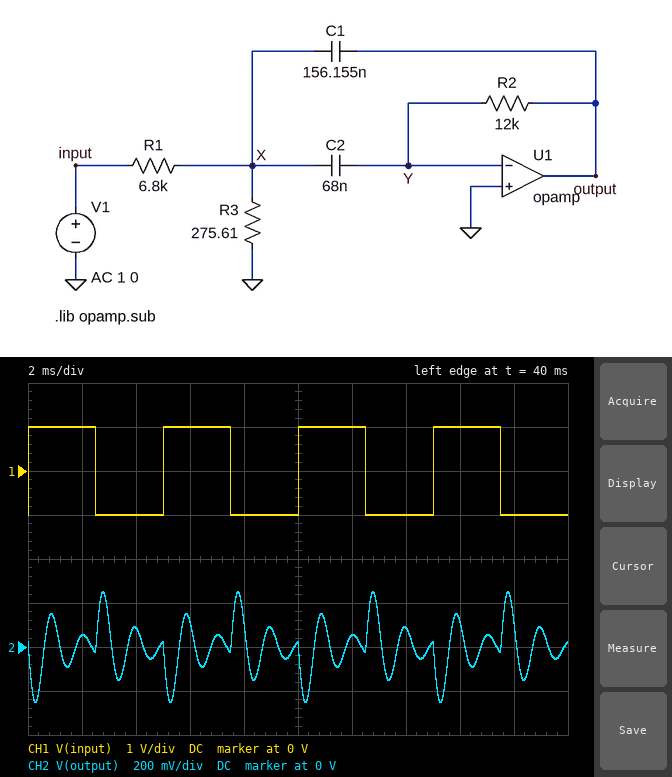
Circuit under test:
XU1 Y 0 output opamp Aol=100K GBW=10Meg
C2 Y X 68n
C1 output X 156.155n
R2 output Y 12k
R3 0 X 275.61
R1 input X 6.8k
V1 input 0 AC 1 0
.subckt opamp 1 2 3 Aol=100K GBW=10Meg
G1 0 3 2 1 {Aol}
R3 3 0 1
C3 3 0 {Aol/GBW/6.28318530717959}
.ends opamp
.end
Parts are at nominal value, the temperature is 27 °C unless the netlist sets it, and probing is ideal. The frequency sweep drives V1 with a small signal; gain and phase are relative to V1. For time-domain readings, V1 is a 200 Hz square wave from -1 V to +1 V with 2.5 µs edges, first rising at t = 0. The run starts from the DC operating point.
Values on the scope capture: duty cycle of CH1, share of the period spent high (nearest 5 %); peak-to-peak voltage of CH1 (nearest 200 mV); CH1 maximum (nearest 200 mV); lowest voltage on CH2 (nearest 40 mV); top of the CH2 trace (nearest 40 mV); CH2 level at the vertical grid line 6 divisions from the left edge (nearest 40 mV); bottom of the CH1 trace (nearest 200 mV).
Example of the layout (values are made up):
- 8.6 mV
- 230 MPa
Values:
- 50 %
- 2.0 V
- 1.0 V
- -240 mV
- 240 mV
- 40 mV
- -1.0 V
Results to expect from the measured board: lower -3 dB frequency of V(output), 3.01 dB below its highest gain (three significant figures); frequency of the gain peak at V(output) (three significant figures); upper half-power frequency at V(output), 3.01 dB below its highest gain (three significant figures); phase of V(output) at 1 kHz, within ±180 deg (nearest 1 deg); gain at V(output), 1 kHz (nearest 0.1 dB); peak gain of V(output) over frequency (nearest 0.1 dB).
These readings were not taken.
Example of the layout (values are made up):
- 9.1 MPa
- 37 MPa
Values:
- 737 Hz
- 866 Hz
- 1.02 kHz
- 138 deg
- -8.0 dB
- -5.4 dB
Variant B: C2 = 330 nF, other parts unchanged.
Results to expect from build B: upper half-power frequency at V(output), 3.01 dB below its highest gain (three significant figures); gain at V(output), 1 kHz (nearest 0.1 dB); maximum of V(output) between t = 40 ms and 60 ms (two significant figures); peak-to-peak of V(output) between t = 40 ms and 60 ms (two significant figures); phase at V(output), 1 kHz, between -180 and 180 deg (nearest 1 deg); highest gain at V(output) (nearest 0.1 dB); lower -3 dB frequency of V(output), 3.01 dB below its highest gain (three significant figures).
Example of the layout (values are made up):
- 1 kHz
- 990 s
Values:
- 461 Hz
- -15.1 dB
- 450 mV
- 890 mV
- 98 deg
- 1.6 dB
- 336 Hz
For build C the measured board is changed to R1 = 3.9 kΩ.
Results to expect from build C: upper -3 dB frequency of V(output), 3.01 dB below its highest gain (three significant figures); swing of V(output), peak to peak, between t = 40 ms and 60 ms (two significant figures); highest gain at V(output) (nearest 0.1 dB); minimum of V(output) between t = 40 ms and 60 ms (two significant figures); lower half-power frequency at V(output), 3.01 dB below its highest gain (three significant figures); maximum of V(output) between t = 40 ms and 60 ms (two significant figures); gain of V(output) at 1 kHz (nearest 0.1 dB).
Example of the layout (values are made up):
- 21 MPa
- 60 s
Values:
- 1.03 kHz
- 880 mV
- -0.6 dB
- -440 mV
- 750 Hz
- 440 mV
- -2.8 dB
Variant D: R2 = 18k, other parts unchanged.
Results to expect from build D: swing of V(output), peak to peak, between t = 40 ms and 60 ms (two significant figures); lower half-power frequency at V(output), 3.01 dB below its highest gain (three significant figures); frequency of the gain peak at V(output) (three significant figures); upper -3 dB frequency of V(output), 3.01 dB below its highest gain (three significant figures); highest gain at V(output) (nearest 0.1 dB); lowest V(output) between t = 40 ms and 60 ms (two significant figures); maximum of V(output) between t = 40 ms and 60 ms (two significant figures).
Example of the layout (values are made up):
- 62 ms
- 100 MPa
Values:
- 700 mV
- 620 Hz
- 707 Hz
- 807 Hz
- -1.9 dB
- -350 mV
- 350 mV
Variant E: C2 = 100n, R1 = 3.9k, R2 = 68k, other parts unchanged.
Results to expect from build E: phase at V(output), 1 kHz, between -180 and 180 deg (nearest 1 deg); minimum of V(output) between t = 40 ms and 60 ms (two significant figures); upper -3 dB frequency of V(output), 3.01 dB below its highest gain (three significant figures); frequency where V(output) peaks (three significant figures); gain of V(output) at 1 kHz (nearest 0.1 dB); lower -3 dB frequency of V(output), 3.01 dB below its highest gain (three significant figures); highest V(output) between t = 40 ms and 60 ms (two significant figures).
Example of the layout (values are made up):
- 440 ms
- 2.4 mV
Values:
- 92 deg
- -1.3 V
- 324 Hz
- 304 Hz
- -10.8 dB
- 286 Hz
- 1.3 V
